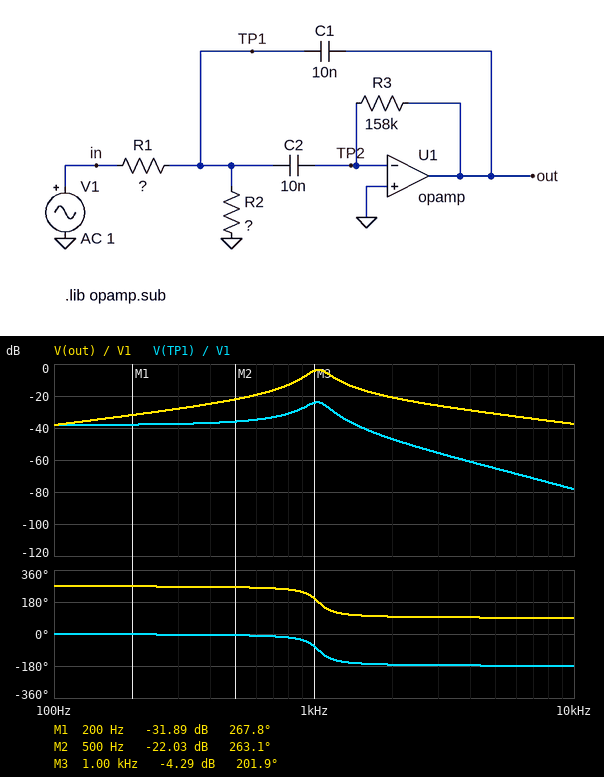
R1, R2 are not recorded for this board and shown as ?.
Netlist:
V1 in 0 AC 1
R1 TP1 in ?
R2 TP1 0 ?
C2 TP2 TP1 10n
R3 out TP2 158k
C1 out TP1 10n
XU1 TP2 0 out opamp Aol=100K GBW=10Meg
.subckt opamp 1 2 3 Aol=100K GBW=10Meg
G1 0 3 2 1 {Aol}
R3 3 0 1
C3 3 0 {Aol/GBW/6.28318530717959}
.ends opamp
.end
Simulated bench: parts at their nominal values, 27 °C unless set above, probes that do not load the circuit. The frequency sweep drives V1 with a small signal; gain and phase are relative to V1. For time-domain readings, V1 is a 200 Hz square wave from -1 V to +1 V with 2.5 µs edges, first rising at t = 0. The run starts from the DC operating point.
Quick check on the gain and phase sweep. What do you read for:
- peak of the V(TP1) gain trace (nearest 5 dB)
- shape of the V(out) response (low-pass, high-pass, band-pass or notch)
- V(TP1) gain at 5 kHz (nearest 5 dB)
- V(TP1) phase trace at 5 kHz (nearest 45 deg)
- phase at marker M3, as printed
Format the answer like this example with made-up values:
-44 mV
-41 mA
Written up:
-25 dB
band-pass
-65 dB
-180 deg
201.9 deg
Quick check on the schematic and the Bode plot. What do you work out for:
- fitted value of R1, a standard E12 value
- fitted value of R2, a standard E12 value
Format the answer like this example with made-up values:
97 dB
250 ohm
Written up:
120 kΩ
1.5 kΩ
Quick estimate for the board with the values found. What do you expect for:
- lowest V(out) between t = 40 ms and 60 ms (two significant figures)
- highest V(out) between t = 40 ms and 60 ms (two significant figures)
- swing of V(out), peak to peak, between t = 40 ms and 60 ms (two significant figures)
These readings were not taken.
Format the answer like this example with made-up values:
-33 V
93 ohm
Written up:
-270 mV
270 mV
540 mV
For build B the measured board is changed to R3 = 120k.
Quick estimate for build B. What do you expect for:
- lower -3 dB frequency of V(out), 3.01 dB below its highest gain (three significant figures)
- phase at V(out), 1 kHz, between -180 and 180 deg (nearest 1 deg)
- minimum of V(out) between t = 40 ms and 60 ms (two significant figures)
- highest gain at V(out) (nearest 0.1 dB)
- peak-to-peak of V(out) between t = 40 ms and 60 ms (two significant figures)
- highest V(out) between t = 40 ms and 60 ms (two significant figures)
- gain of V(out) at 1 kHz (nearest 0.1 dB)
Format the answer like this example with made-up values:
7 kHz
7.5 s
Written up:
1.07 kHz
-122 deg
-170 mV
-6.0 dB
340 mV
170 mV
-11.5 dB
